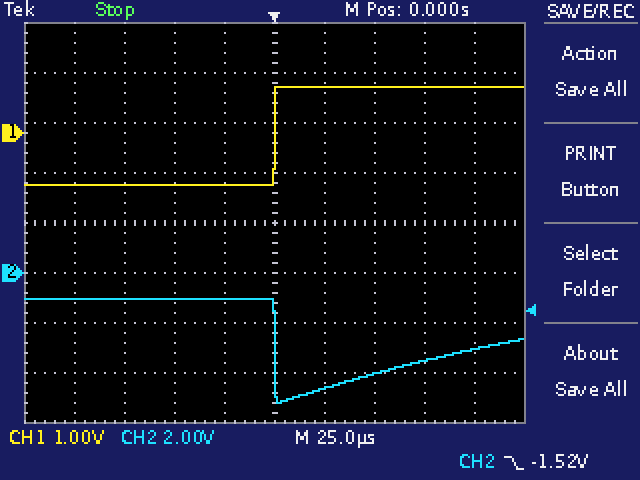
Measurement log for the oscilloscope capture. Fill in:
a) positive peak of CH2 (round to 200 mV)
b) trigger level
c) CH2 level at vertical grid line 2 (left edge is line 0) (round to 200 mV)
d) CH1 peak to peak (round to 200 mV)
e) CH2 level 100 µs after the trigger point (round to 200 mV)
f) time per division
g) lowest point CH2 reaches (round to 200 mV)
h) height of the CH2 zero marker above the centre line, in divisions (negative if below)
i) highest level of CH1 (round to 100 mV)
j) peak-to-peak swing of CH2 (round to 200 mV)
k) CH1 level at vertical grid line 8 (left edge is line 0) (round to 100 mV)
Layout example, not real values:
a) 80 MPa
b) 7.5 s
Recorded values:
a) -1.0 V
b) -1.52 V
c) -1.0 V
d) 2.0 V
e) -3.0 V
f) 25 µs
g) -5.2 V
h) -1.0 div
i) 900 mV
j) 4.2 V
k) 900 mV
